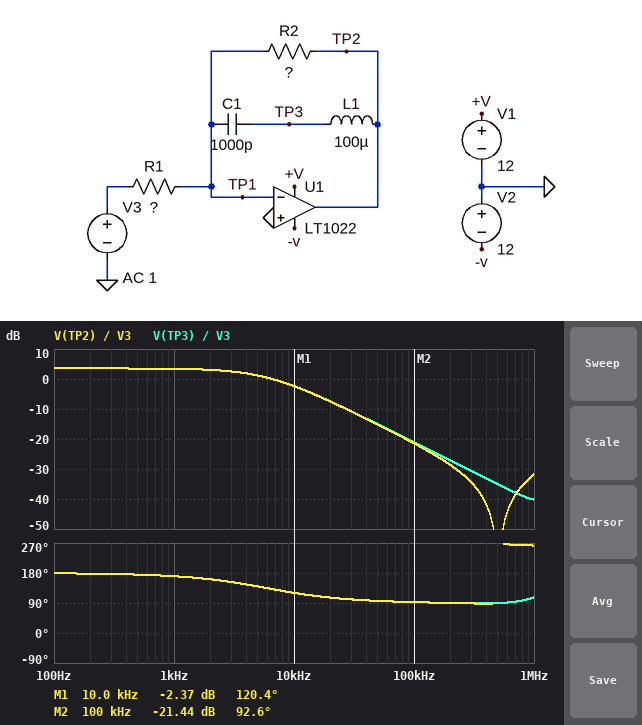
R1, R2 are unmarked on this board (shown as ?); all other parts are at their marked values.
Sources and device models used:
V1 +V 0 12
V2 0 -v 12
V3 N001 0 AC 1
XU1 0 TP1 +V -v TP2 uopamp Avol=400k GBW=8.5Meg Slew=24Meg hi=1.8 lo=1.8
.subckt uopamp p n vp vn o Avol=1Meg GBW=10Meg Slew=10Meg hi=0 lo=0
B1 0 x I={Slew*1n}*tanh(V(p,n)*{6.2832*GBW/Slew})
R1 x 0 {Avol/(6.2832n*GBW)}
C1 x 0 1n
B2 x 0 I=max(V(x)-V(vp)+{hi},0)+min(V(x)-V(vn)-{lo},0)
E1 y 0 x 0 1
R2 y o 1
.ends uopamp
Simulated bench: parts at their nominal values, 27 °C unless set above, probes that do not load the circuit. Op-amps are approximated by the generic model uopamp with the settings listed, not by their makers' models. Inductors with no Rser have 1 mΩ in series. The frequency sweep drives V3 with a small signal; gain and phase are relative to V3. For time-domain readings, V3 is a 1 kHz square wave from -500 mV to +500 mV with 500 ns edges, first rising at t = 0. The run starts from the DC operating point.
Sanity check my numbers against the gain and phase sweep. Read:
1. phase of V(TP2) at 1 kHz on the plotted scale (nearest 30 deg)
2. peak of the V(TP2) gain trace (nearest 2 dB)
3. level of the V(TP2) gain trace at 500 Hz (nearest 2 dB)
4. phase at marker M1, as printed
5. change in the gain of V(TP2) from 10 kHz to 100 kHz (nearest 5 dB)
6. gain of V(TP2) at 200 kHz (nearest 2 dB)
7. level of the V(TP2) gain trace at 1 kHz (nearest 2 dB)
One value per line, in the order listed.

180 deg
4 dB
4 dB
120.4 deg
-20 dB
-28 dB
4 dB
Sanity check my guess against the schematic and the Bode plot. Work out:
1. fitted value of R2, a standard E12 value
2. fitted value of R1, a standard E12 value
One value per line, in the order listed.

27 kΩ
18 kΩ
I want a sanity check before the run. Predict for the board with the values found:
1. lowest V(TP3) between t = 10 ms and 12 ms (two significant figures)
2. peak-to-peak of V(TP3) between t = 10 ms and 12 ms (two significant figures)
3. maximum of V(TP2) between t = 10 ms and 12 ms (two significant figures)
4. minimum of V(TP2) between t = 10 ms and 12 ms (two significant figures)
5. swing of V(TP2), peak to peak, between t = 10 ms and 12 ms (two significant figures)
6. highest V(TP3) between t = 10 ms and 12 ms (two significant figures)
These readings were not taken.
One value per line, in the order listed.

-760 mV
1.5 V
750 mV
-750 mV
1.5 V
760 mV
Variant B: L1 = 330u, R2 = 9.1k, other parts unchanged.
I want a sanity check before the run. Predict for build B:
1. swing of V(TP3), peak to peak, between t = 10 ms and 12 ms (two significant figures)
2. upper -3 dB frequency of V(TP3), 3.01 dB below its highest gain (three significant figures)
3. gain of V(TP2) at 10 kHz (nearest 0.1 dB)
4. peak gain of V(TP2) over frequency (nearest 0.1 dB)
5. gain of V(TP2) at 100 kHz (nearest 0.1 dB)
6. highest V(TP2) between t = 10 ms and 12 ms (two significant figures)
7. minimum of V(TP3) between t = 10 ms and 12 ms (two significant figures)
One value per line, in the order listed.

520 mV
17.5 kHz
-7.2 dB
-5.9 dB
-22.4 dB
250 mV
-260 mV
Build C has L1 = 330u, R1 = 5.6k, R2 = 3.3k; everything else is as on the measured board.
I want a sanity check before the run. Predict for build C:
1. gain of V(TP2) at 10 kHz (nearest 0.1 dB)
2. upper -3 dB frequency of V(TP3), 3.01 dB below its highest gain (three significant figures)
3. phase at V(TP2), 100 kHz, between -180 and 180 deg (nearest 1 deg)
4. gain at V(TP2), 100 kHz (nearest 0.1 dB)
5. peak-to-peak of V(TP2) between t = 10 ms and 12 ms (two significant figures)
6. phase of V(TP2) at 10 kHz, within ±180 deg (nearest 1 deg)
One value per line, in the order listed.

-4.8 dB
49.6 kHz
112 deg
-12.9 dB
590 mV
168 deg
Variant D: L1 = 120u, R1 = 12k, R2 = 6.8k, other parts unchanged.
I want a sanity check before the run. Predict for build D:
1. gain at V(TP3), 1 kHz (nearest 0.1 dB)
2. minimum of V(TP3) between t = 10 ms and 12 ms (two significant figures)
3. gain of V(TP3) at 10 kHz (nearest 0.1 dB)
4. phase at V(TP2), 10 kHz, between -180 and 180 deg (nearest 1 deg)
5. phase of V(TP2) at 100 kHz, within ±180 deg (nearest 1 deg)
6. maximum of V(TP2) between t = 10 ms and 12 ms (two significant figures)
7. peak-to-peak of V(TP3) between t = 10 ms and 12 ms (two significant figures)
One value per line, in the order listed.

-4.9 dB
-290 mV
-5.7 dB
157 deg
102 deg
280 mV
580 mV
